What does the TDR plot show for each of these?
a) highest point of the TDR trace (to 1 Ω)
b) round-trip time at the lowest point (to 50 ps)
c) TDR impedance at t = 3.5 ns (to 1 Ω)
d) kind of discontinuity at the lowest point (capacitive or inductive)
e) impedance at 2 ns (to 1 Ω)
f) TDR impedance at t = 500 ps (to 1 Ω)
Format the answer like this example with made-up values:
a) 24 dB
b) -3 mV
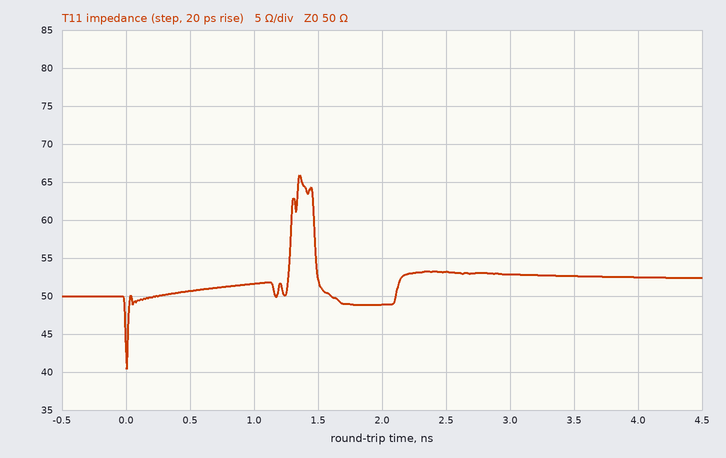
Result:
a) 66 Ω
b) 0 ps
c) 53 Ω
d) capacitive
e) 49 Ω
f) 51 Ω
